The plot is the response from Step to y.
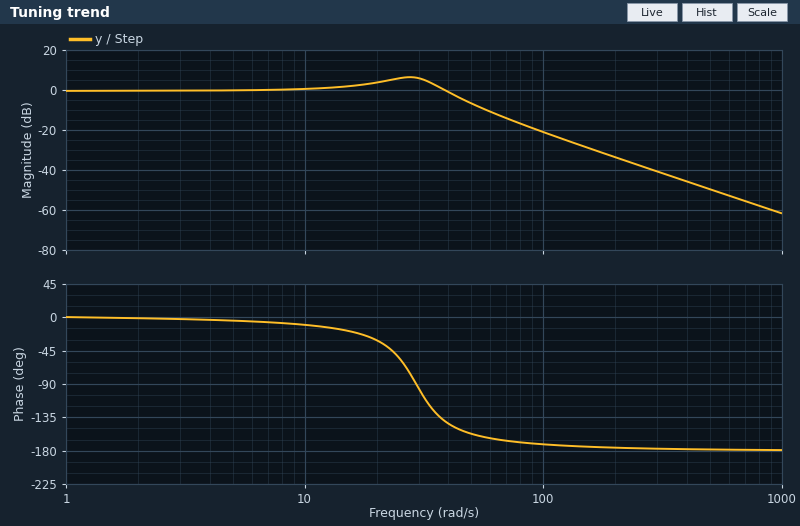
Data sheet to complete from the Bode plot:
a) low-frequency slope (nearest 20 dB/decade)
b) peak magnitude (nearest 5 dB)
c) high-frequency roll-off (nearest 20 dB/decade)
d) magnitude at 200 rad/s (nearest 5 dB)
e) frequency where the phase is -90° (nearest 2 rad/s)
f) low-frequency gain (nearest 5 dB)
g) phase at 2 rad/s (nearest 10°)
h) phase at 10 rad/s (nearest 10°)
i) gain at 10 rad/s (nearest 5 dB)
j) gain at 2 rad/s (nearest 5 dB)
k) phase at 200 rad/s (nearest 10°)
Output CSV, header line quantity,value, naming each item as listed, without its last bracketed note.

quantity,value
low-frequency slope,0 dB/decade
peak magnitude,5 dB
high-frequency roll-off,-40 dB/decade
magnitude at 200 rad/s,-35 dB
frequency where the phase is -90°,30 rad/s
low-frequency gain,0 dB
phase at 2 rad/s,0°
phase at 10 rad/s,-10°
gain at 10 rad/s,0 dB
gain at 2 rad/s,0 dB
phase at 200 rad/s,-180°
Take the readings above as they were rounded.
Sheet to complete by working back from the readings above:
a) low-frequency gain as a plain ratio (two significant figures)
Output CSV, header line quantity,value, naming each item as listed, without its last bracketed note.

quantity,value
low-frequency gain as a plain ratio,1.0
